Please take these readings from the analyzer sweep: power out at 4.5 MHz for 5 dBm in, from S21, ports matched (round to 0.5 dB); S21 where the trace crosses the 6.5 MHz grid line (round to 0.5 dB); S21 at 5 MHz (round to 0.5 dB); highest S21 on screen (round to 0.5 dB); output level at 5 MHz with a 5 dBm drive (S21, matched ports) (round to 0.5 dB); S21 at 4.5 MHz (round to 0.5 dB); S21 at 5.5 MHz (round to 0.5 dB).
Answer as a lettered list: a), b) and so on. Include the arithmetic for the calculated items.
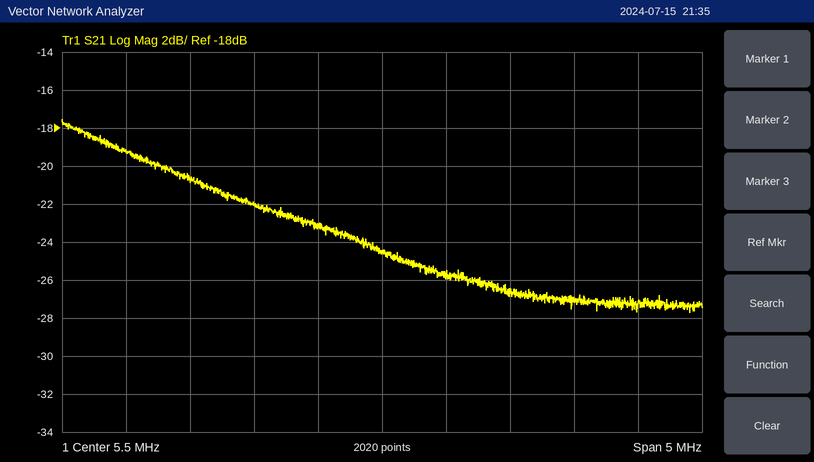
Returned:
a) 5 dBm + (-22.0 dB) = -17.0 dBm
b) -26.5 dB
c) -23.0 dB
d) -17.5 dB
e) 5 dBm + (-23.0 dB) = -18.0 dBm
f) -22.0 dB
g) -24.5 dB
